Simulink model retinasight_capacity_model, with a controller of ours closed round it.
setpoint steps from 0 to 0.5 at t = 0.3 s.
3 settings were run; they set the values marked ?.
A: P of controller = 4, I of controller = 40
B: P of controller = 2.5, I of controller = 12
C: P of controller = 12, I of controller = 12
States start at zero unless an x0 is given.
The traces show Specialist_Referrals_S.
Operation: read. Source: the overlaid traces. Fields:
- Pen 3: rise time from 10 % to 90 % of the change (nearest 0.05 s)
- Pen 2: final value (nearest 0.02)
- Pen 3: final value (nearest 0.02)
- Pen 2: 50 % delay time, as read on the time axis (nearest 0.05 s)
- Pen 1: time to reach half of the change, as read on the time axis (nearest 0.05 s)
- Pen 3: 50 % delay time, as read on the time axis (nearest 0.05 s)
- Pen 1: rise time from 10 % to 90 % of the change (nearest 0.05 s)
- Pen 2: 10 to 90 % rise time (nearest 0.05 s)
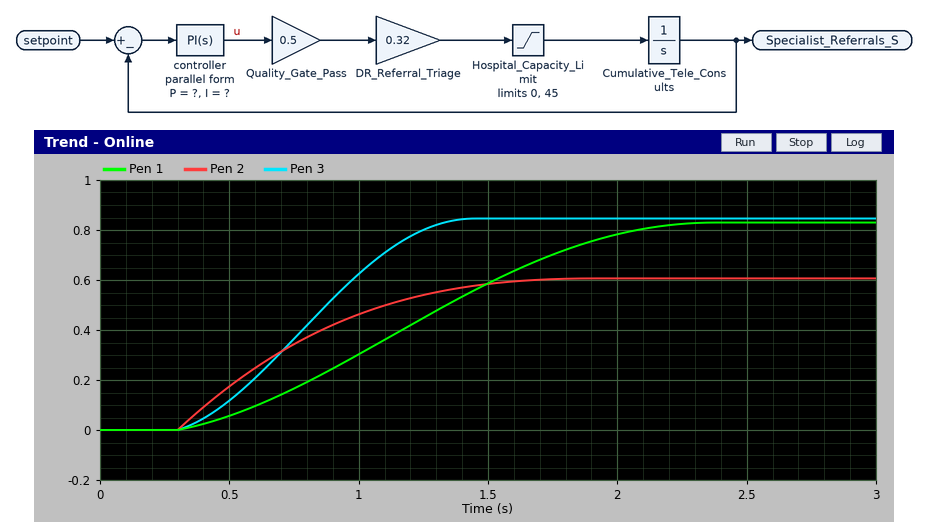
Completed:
0.70 s
0.60
0.84
0.70 s
1.20 s
0.80 s
1.30 s
0.90 s
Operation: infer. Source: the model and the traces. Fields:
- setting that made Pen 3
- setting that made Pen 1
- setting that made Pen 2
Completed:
A
B
C
